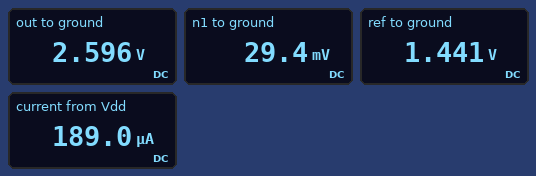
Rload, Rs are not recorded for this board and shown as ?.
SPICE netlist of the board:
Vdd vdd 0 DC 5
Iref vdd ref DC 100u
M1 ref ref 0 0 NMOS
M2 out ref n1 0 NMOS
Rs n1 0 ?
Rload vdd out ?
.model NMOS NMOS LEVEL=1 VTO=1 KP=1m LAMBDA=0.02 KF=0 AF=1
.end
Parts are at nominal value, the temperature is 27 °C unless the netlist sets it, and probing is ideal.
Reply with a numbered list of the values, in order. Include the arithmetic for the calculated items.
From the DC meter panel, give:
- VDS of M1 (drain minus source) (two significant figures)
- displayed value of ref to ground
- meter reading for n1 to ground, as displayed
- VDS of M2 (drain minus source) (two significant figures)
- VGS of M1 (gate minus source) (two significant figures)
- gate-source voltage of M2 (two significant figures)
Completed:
1. 1.441 V = 1.4 V
2. 1.441 V
3. 29.4 mV
4. 2.596 V - 29.4 mV = 2.6 V
5. 1.441 V = 1.4 V
6. 1.441 V - 29.4 mV = 1.4 V
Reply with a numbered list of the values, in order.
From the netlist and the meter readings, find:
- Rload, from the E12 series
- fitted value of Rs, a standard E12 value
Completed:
1. 27 kΩ
2. 330 Ω
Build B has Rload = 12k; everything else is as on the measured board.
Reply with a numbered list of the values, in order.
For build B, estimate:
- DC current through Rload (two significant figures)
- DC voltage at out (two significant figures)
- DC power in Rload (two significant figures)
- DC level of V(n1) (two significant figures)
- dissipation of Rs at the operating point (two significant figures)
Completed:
1. 91 µA
2. 3.9 V
3. 99 µW
4. 30 mV
5. 2.7 µW
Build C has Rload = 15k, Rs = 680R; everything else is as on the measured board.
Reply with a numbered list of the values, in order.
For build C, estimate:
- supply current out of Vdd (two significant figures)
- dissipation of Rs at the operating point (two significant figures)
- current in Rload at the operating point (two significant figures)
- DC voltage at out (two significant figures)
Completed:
1. 180 µA
2. 4.4 µW
3. 80 µA
4. 3.8 V
